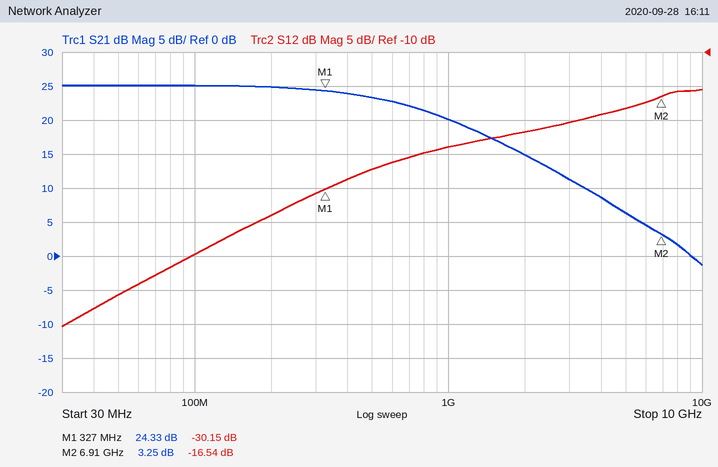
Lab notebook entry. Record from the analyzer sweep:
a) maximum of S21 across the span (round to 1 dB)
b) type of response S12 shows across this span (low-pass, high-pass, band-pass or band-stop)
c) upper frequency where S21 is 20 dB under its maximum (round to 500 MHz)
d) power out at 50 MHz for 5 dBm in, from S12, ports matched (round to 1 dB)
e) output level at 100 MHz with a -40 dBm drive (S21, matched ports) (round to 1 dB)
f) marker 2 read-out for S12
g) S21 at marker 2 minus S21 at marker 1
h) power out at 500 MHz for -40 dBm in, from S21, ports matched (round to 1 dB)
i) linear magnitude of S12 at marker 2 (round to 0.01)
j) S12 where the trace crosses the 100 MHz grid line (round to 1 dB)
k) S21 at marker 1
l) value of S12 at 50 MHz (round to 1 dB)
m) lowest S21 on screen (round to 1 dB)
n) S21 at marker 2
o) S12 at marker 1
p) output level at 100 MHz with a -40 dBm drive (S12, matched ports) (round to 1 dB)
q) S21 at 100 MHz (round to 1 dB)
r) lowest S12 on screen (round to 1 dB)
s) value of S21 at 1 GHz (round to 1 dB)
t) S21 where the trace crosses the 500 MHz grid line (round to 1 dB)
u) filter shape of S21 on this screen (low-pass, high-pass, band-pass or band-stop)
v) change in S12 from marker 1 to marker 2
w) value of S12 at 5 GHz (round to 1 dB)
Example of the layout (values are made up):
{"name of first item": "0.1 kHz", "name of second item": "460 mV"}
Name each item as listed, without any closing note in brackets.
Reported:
{"maximum of S21 across the span": "25 dB", "type of response S12 shows across this span": "high-pass", "upper frequency where S21 is 20 dB under its maximum": "5.5 GHz", "power out at 50 MHz for 5 dBm in, from S12, ports matched": "-41 dBm", "output level at 100 MHz with a -40 dBm drive (S21, matched ports)": "-15 dBm", "marker 2 read-out for S12": "-16.54 dB", "S21 at marker 2 minus S21 at marker 1": "-21.08 dB", "power out at 500 MHz for -40 dBm in, from S21, ports matched": "-17 dBm", "linear magnitude of S12 at marker 2": "0.15", "S12 where the trace crosses the 100 MHz grid line": "-40 dB", "S21 at marker 1": "24.33 dB", "value of S12 at 50 MHz": "-46 dB", "lowest S21 on screen": "-1 dB", "S21 at marker 2": "3.25 dB", "S12 at marker 1": "-30.15 dB", "output level at 100 MHz with a -40 dBm drive (S12, matched ports)": "-80 dBm", "S21 at 100 MHz": "25 dB", "lowest S12 on screen": "-50 dB", "value of S21 at 1 GHz": "20 dB", "S21 where the trace crosses the 500 MHz grid line": "23 dB", "filter shape of S21 on this screen": "low-pass", "change in S12 from marker 1 to marker 2": "13.61 dB", "value of S12 at 5 GHz": "-18 dB"}
